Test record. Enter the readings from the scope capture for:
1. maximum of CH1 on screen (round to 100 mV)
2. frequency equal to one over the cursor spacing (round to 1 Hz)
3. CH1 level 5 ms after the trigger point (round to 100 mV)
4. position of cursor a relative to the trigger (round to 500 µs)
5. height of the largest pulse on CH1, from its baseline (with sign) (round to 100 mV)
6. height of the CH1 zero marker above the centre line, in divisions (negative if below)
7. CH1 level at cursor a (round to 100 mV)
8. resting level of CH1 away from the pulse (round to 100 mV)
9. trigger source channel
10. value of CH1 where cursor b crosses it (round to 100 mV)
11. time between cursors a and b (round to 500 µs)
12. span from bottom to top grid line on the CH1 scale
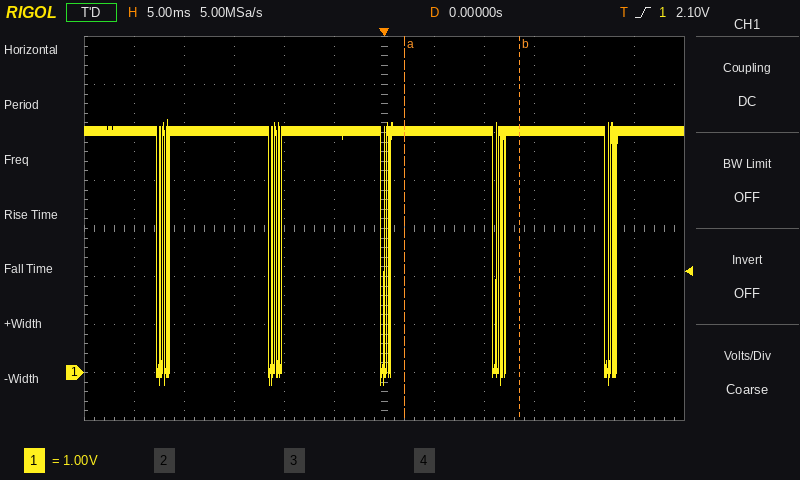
5.3 V
87 Hz
5.0 V
+2.0 ms
-5.3 V
-3.0 div
5.0 V
5.0 V
CH1
5.0 V
11.5 ms
8 V
